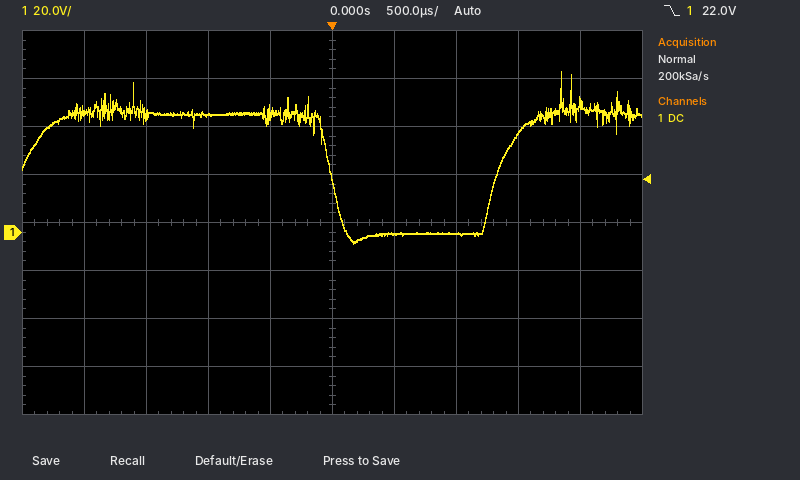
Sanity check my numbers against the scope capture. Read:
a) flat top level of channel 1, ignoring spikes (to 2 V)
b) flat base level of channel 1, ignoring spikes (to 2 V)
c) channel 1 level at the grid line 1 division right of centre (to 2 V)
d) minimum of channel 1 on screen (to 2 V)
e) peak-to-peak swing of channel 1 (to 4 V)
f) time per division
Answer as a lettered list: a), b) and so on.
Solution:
a) 50 V
b) 0 V
c) 0 V
d) -4 V
e) 72 V
f) 500 µs
